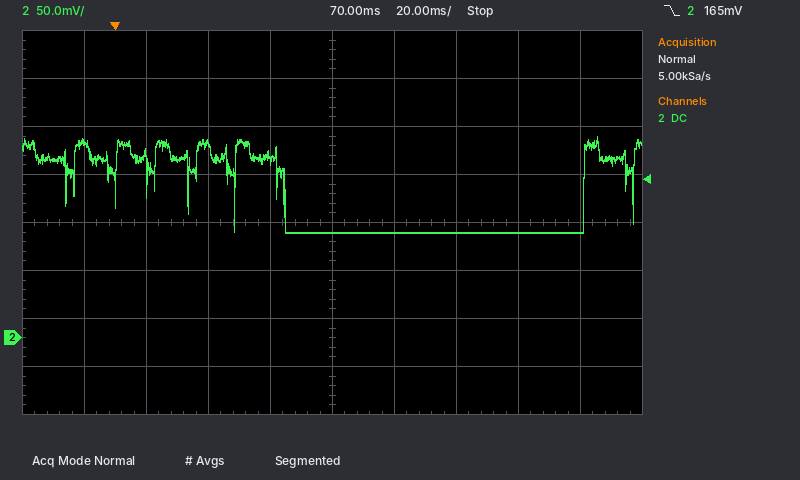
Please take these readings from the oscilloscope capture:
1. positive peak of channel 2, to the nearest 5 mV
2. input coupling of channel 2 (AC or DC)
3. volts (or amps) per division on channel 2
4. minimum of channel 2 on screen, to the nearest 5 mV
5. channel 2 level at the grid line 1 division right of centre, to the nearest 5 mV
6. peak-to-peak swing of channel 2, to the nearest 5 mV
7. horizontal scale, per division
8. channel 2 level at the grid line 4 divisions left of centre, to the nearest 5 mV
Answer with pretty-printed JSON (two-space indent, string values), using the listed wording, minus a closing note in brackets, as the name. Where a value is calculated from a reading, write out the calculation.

{
  "positive peak of channel 2, to the nearest 5 mV": "210 mV",
  "input coupling of channel 2": "DC",
  "volts (or amps) per division on channel 2": "50 mV",
  "minimum of channel 2 on screen, to the nearest 5 mV": "110 mV",
  "channel 2 level at the grid line 1 division right of centre, to the nearest 5 mV": "110 mV",
  "peak-to-peak swing of channel 2, to the nearest 5 mV": "210 mV − (110 mV) = 100 mV",
  "horizontal scale, per division": "20 ms",
  "channel 2 level at the grid line 4 divisions left of centre, to the nearest 5 mV": "205 mV"
}
